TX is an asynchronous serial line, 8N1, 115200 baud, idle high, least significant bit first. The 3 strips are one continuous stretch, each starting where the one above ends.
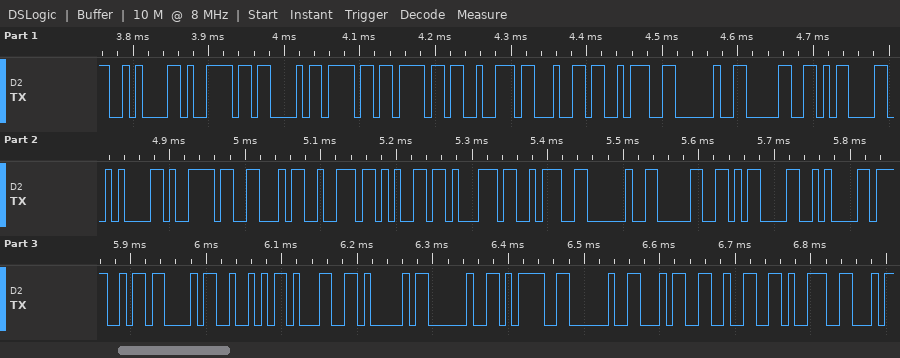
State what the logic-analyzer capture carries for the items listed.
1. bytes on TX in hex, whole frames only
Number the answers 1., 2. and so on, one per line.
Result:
1. 0A 79 43 6F 6F 72 64 3A 20 30 0D 0A 79 46 72 65 71 3A 20 30 0D 0A 4F 43 52 31 41 20 3D 20 34 32 39
